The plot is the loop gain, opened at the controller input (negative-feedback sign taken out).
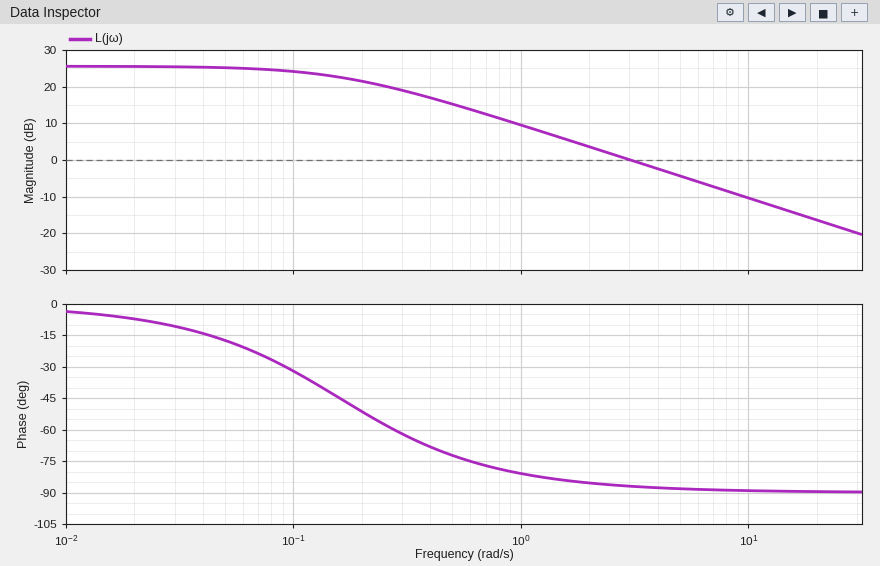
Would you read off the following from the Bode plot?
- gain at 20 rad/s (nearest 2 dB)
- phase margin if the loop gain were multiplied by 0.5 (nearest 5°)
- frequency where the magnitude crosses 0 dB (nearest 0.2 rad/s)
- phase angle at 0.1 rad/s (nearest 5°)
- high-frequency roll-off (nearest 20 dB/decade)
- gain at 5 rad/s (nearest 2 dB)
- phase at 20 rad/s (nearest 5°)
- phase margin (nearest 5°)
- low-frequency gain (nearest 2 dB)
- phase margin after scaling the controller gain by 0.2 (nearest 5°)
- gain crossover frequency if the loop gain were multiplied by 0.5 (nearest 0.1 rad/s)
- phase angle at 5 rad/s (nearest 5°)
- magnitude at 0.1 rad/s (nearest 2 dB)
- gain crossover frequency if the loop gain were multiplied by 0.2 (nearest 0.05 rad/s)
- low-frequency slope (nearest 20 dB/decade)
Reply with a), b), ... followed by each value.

a) -16 dB
b) 95°
c) 3.0 rad/s
d) -30°
e) -20 dB/decade
f) -4 dB
g) -90°
h) 95°
i) 26 dB
j) 105°
k) 1.5 rad/s
l) -90°
m) 24 dB
n) 0.60 rad/s
o) 0 dB/decade
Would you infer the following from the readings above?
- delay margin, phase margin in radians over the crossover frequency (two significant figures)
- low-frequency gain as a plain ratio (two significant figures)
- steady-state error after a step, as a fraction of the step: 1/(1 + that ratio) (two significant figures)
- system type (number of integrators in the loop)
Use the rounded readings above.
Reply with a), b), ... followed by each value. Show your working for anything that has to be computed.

a) 95 × π / 180 / 3 = 0.55 s
b) 10^(26 / 20) = 20
c) 1 / (1 + 20) = 0.048
d) 0
